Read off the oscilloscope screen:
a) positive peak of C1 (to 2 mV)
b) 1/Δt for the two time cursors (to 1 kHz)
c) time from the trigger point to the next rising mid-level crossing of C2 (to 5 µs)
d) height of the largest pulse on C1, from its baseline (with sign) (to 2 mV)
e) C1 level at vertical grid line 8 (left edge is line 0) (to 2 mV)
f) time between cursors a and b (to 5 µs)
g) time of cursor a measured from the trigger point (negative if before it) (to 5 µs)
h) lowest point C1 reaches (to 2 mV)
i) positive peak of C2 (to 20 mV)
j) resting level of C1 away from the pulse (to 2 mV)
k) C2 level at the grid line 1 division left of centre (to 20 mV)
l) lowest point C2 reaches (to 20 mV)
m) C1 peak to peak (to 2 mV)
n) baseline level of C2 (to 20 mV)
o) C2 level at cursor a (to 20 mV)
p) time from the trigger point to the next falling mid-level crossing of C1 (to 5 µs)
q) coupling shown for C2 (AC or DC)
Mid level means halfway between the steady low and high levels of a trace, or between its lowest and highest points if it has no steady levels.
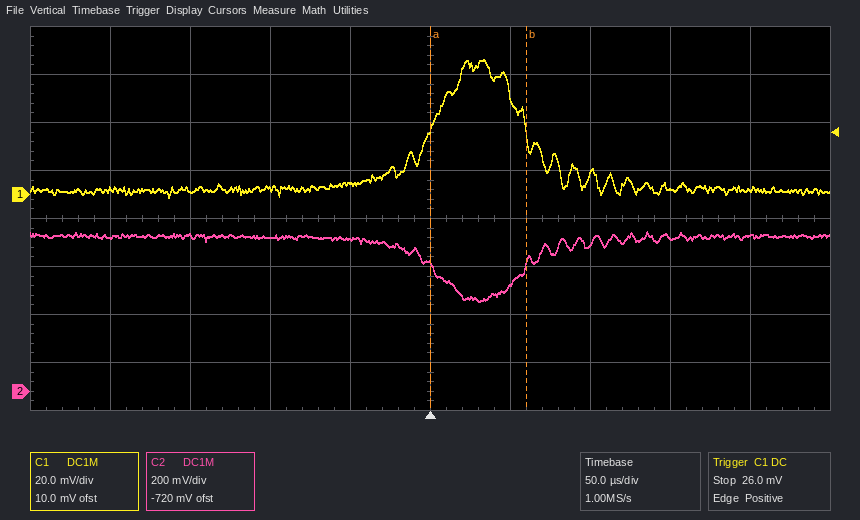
56 mV
17 kHz
60 µs
+54 mV
2 mV
60 µs
0 µs
-2 mV
660 mV
2 mV
640 mV
380 mV
58 mV
640 mV
520 mV
60 µs
DC
